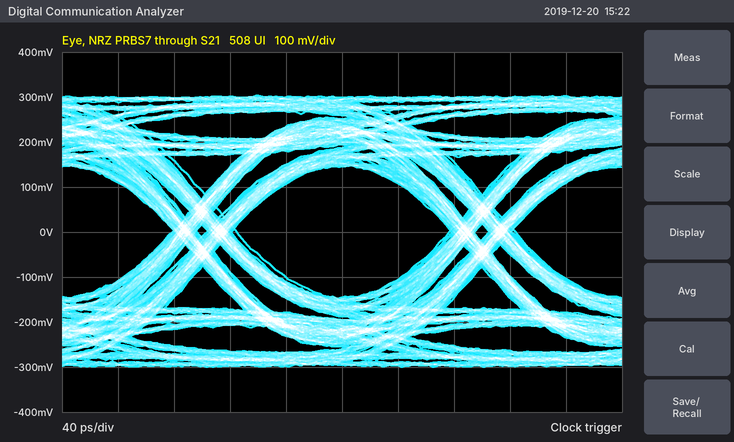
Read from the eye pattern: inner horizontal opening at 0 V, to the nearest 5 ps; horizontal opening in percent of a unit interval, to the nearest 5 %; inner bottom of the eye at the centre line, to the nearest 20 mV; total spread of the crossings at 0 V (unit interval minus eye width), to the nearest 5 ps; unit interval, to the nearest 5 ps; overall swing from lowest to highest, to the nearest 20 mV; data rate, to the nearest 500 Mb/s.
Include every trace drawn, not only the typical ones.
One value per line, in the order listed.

150 ps
75 %
-140 mV
50 ps
200 ps
600 mV
5.0 Gb/s
